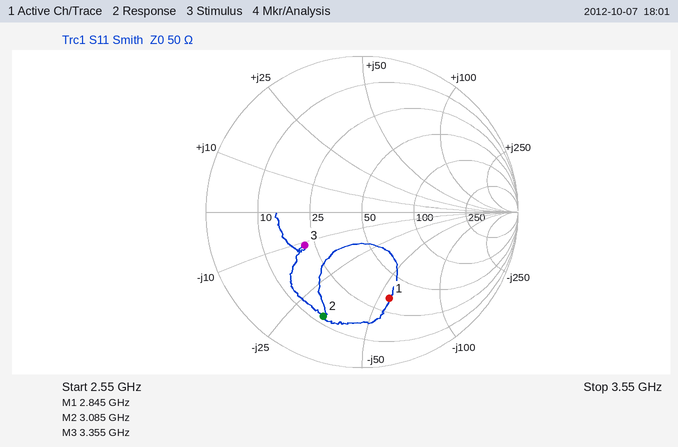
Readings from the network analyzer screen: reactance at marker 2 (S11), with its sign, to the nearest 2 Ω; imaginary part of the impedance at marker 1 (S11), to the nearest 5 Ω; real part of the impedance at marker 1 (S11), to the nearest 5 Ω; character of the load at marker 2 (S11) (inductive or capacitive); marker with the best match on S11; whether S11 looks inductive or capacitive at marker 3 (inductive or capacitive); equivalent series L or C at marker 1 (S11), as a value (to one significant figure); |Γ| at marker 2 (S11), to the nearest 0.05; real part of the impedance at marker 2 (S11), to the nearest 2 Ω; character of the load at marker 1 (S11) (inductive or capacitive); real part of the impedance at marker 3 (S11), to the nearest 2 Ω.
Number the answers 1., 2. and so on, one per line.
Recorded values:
1. -34 Ω
2. -55 Ω
3. 35 Ω
4. capacitive
5. marker 3
6. capacitive
7. 1.0 pF
8. 0.70
9. 12 Ω
10. capacitive
11. 22 Ω
